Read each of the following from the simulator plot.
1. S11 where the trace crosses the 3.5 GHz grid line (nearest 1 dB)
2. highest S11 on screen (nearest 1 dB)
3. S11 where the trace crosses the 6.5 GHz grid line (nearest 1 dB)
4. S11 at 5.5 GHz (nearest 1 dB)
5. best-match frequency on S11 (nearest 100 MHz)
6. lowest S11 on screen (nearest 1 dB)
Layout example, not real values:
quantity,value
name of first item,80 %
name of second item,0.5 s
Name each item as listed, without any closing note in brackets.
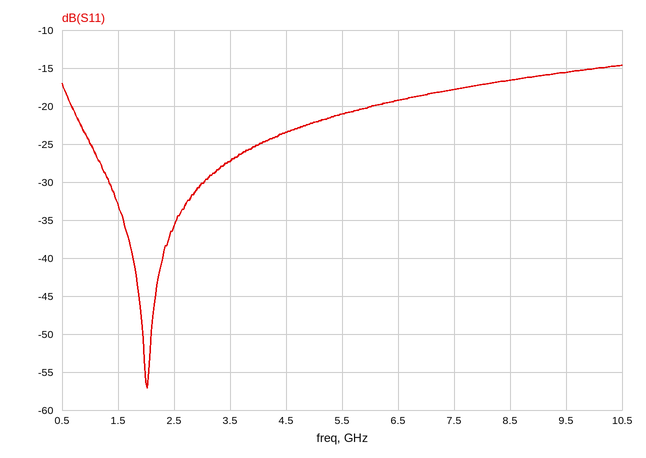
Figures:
quantity,value
S11 where the trace crosses the 3.5 GHz grid line,-27 dB
highest S11 on screen,-15 dB
S11 where the trace crosses the 6.5 GHz grid line,-19 dB
S11 at 5.5 GHz,-21 dB
best-match frequency on S11,2.0 GHz
lowest S11 on screen,-57 dB
